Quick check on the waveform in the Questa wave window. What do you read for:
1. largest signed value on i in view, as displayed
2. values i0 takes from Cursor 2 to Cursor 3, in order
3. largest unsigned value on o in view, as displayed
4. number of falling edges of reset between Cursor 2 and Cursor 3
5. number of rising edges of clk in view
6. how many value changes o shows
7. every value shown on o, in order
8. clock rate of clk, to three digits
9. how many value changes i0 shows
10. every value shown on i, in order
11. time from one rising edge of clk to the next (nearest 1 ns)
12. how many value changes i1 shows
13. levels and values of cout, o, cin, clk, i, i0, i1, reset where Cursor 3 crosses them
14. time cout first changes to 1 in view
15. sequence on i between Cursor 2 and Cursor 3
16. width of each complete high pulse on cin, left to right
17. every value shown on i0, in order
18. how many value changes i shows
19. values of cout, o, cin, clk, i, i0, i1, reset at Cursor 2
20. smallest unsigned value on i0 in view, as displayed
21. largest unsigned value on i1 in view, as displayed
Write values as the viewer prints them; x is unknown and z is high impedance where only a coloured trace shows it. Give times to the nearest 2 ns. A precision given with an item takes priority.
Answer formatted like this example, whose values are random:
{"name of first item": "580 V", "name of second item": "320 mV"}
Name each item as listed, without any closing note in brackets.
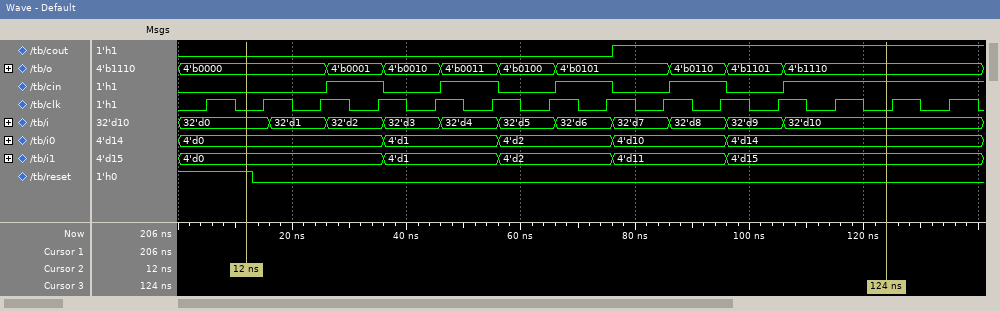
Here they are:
{"largest signed value on i in view, as displayed": "32'd10", "values i0 takes from Cursor 2 to Cursor 3, in order": "4'd0, 4'd1, 4'd2, 4'd10, 4'd14", "largest unsigned value on o in view, as displayed": "4'b1110", "number of falling edges of reset between Cursor 2 and Cursor 3": "1", "number of rising edges of clk in view": "14", "how many value changes o shows": "8", "every value shown on o, in order": "4'b0000, 4'b0001, 4'b0010, 4'b0011, 4'b0100, 4'b0101, 4'b0110, 4'b1101, 4'b1110", "clock rate of clk, to three digits": "100 MHz", "how many value changes i0 shows": "4", "every value shown on i, in order": "32'd0, 32'd1, 32'd2, 32'd3, 32'd4, 32'd5, 32'd6, 32'd7, 32'd8, 32'd9, 32'd10", "time from one rising edge of clk to the next": "10 ns", "how many value changes i1 shows": "4", "levels and values of cout, o, cin, clk, i, i0, i1, reset where Cursor 3 crosses them": "cout=1, o=4'b1110, cin=1, clk=0, i=32'd10, i0=4'd14, i1=4'd15, reset=0", "time cout first changes to 1 in view": "76 ns", "sequence on i between Cursor 2 and Cursor 3": "32'd0, 32'd1, 32'd2, 32'd3, 32'd4, 32'd5, 32'd6, 32'd7, 32'd8, 32'd9, 32'd10", "width of each complete high pulse on cin, left to right": "10 ns, 10 ns, 10 ns, 10 ns", "every value shown on i0, in order": "4'd0, 4'd1, 4'd2, 4'd10, 4'd14", "how many value changes i shows": "10", "values of cout, o, cin, clk, i, i0, i1, reset at Cursor 2": "cout=0, o=4'b0000, cin=0, clk=0, i=32'd0, i0=4'd0, i1=4'd0, reset=1", "smallest unsigned value on i0 in view, as displayed": "4'd0", "largest unsigned value on i1 in view, as displayed": "4'd15"}
